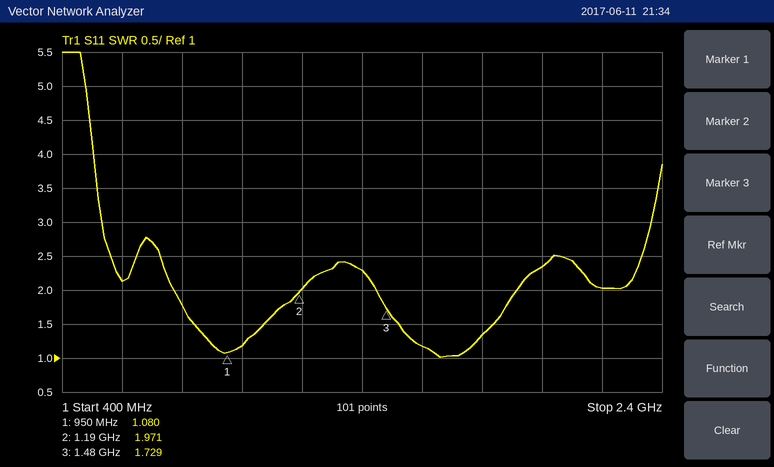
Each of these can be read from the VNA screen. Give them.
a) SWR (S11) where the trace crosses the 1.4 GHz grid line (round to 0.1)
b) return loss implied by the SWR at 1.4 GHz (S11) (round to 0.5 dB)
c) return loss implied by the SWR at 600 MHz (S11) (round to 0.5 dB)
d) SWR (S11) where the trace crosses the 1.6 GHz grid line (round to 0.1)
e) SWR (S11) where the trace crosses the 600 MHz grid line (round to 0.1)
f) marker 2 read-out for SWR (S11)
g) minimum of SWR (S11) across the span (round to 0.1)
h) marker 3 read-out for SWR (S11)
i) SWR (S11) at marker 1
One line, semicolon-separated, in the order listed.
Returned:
2.3; 8.0 dB; 9.0 dB; 1.2; 2.1; 1.971; 1.0; 1.729; 1.080
